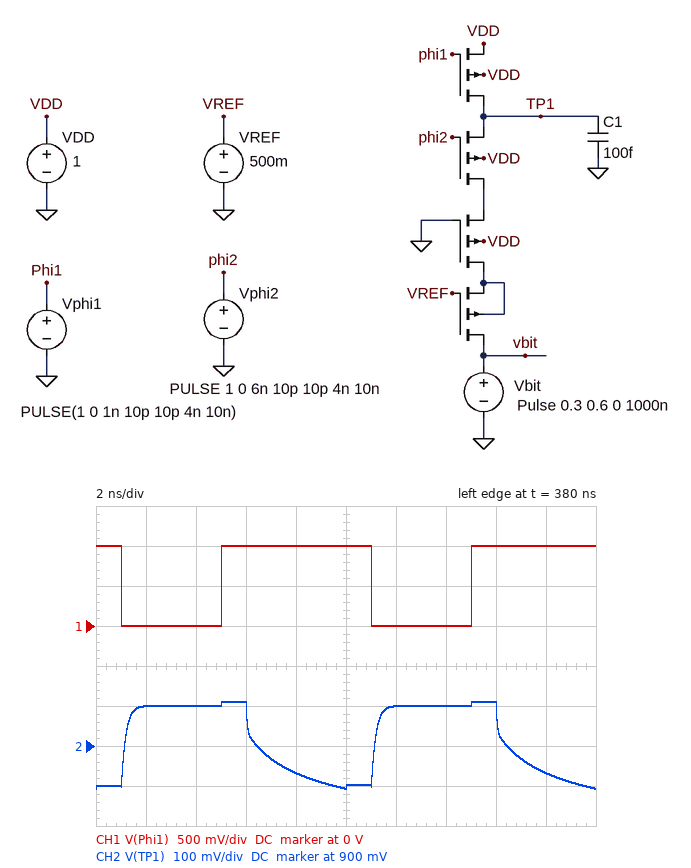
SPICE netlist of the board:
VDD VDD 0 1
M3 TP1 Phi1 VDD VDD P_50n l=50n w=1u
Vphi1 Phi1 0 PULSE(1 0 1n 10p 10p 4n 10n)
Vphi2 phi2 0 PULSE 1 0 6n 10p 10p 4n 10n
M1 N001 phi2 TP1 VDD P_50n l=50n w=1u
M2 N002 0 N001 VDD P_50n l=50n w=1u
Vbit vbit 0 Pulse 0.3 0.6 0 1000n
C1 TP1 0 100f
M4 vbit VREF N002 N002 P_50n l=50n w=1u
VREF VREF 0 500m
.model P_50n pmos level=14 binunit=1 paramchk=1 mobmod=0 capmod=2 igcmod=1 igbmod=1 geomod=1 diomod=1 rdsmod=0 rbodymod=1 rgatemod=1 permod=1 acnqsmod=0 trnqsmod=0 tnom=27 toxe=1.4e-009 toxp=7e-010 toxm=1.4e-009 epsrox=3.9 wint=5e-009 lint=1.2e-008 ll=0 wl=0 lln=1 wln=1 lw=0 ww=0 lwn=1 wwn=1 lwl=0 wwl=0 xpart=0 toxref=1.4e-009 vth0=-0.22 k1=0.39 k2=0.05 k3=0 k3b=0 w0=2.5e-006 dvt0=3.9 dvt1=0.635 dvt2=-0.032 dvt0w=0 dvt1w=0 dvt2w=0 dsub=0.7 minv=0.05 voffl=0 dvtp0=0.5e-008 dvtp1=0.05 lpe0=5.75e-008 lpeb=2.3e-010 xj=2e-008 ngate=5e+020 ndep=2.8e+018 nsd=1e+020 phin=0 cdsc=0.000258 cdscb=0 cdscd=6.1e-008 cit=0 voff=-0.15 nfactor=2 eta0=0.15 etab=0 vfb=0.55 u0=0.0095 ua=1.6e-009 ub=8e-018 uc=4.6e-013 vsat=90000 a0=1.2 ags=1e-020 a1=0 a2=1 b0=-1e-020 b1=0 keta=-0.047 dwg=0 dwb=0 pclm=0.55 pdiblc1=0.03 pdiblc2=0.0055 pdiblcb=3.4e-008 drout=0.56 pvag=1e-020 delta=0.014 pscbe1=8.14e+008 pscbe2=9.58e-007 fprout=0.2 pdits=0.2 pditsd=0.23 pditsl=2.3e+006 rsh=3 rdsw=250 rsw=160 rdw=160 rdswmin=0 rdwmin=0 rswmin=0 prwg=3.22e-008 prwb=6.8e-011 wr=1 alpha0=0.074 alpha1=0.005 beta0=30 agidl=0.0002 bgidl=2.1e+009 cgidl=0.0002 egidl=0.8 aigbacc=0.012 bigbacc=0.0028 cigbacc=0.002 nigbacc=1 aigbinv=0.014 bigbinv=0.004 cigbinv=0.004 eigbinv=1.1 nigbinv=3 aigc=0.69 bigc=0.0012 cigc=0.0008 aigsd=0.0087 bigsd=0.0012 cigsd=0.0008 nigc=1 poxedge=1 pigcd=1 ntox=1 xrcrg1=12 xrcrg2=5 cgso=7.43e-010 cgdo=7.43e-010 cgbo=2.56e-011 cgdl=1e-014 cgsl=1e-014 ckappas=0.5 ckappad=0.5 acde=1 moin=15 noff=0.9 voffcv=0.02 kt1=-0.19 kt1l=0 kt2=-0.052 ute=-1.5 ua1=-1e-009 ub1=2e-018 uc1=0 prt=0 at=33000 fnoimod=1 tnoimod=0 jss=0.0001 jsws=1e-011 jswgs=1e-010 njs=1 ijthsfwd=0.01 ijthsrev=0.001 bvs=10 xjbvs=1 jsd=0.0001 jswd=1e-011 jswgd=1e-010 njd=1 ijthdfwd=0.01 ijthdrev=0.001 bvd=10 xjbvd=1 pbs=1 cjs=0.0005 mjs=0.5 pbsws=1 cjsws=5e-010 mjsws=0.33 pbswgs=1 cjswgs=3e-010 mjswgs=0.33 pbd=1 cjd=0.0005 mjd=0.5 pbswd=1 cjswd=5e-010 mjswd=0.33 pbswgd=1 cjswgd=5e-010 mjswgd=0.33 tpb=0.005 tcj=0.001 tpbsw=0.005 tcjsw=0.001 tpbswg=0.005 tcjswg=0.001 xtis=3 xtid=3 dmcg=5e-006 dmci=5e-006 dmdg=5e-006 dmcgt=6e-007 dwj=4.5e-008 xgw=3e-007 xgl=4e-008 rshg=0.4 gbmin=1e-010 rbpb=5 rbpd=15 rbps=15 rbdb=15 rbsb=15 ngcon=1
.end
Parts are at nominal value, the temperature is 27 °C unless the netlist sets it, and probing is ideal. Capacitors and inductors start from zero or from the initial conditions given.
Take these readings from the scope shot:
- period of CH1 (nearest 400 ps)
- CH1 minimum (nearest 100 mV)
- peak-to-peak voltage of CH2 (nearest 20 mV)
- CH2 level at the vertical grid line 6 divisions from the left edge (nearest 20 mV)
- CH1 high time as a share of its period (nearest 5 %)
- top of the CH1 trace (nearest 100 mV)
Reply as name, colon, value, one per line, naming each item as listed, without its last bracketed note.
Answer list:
period of CH1: 10.0 ns
CH1 minimum: 0 V
peak-to-peak voltage of CH2: 220 mV
CH2 level at the vertical grid line 6 divisions from the left edge: 1.00 V
CH1 high time as a share of its period: 60 %
top of the CH1 trace: 1.0 V
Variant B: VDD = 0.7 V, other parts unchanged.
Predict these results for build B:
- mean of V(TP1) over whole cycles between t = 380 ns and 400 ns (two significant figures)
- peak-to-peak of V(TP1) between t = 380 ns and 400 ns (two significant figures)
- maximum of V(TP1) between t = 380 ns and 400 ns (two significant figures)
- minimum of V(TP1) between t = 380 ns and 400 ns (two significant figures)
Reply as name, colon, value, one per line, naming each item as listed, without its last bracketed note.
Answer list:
mean of V(TP1) over whole cycles between t = 380 ns and 400 ns: 690 mV
peak-to-peak of V(TP1) between t = 380 ns and 400 ns: 26 mV
maximum of V(TP1) between t = 380 ns and 400 ns: 710 mV
minimum of V(TP1) between t = 380 ns and 400 ns: 680 mV
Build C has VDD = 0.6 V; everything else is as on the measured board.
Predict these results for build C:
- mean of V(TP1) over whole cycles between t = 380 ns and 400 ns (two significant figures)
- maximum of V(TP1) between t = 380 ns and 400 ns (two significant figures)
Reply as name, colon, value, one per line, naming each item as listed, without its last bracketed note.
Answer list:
mean of V(TP1) over whole cycles between t = 380 ns and 400 ns: 600 mV
maximum of V(TP1) between t = 380 ns and 400 ns: 610 mV
